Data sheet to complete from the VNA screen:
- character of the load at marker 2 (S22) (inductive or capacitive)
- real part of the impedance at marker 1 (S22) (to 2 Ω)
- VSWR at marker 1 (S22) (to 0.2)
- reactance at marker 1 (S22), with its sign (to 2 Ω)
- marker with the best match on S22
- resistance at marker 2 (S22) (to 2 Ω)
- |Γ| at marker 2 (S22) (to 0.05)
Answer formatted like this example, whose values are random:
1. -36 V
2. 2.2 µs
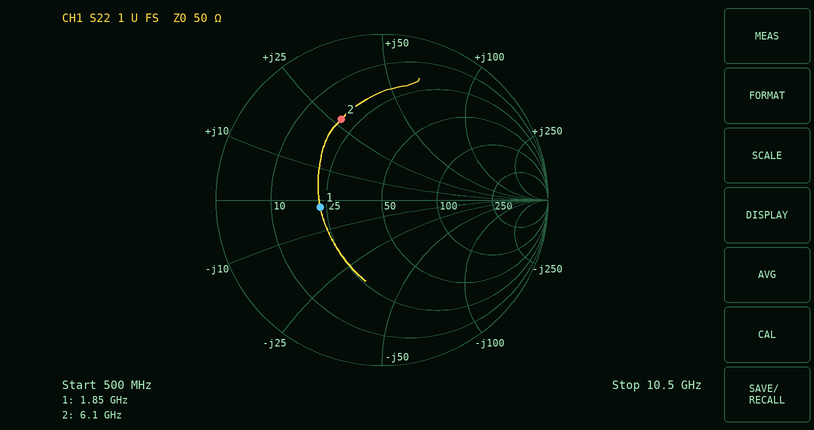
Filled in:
1. inductive
2. 22 Ω
3. 2.2
4. -2 Ω
5. marker 1
6. 20 Ω
7. 0.55
